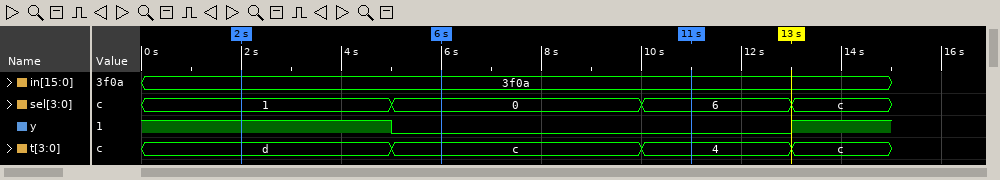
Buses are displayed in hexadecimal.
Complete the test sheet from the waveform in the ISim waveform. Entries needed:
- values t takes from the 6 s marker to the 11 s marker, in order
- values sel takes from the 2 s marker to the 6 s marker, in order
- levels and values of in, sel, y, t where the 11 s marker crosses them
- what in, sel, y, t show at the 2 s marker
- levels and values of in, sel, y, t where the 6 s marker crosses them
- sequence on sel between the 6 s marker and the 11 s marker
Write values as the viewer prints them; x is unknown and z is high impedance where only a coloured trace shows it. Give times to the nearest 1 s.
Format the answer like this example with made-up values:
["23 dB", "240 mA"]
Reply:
["c, 4", "1, 0", "in=3f0a, sel=6, y=0, t=4", "in=3f0a, sel=1, y=1, t=d", "in=3f0a, sel=0, y=0, t=c", "0, 6"]
